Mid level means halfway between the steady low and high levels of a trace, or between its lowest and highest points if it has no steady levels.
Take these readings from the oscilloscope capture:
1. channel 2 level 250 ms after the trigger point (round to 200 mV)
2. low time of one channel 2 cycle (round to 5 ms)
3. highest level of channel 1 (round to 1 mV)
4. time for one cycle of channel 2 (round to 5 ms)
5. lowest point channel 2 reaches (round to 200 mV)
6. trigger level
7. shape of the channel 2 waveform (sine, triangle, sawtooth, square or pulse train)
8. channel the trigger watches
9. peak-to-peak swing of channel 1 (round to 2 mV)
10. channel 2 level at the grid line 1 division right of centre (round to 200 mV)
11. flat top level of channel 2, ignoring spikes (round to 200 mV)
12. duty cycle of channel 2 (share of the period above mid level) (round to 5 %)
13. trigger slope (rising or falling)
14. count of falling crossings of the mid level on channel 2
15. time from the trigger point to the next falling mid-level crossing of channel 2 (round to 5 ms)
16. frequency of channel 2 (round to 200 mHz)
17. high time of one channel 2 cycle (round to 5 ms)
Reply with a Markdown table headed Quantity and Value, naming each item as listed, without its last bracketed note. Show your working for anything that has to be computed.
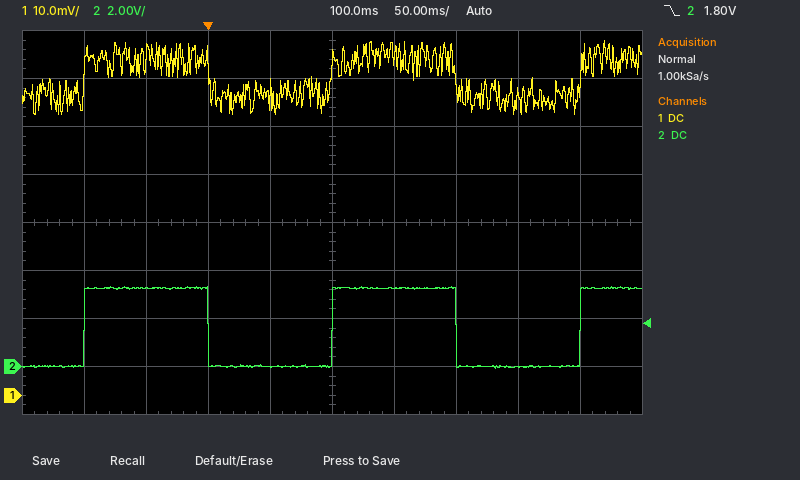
| Quantity | Value |
|---|---|
| channel 2 level 250 ms after the trigger point | 0.0 V |
| low time of one channel 2 cycle | 100 ms |
| highest level of channel 1 | 74 mV |
| time for one cycle of channel 2 | 200 ms |
| lowest point channel 2 reaches | 0.0 V |
| trigger level | 1.80 V |
| shape of the channel 2 waveform | square |
| channel the trigger watches | channel 2 |
| peak-to-peak swing of channel 1 | 16 mV |
| channel 2 level at the grid line 1 division right of centre | 3.2 V |
| flat top level of channel 2, ignoring spikes | 3.2 V |
| duty cycle of channel 2 (share of the period above mid level) | 100 ms / 200 ms ≈ 50 % |
| trigger slope | falling |
| count of falling crossings of the mid level on channel 2 | 2 |
| time from the trigger point to the next falling mid-level crossing of channel 2 | 200 ms |
| frequency of channel 2 | 1 / 200 ms ≈ 5.0 Hz |
| high time of one channel 2 cycle | 100 ms |
